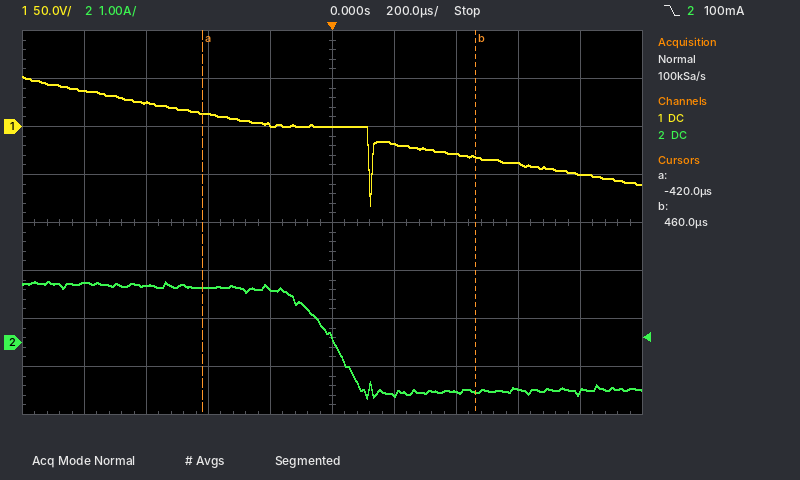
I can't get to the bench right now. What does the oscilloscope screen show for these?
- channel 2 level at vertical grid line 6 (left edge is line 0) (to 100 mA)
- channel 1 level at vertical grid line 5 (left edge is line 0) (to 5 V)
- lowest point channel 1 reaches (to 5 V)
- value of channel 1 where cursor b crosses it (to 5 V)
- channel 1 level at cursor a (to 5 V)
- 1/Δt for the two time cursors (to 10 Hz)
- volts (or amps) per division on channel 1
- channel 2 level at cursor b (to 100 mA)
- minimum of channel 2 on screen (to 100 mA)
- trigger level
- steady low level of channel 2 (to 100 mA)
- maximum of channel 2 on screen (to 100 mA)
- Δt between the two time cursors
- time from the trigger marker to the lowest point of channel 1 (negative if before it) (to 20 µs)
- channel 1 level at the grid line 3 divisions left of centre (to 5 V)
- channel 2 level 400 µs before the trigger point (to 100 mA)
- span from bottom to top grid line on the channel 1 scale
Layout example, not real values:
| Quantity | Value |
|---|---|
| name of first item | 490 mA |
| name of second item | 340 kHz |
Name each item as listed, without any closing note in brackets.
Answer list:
| Quantity | Value |
|---|---|
| channel 2 level at vertical grid line 6 (left edge is line 0) | -1.1 A |
| channel 1 level at vertical grid line 5 (left edge is line 0) | 0 V |
| lowest point channel 1 reaches | -80 V |
| value of channel 1 where cursor b crosses it | -30 V |
| channel 1 level at cursor a | 15 V |
| 1/Δt for the two time cursors | 1.14 kHz |
| volts (or amps) per division on channel 1 | 50 V |
| channel 2 level at cursor b | -1.0 A |
| minimum of channel 2 on screen | -1.2 A |
| trigger level | 100 mA |
| steady low level of channel 2 | -1.0 A |
| maximum of channel 2 on screen | 1.3 A |
| Δt between the two time cursors | 880 µs |
| time from the trigger marker to the lowest point of channel 1 (negative if before it) | +120 µs |
| channel 1 level at the grid line 3 divisions left of centre | 25 V |
| channel 2 level 400 µs before the trigger point | 1.1 A |
| span from bottom to top grid line on the channel 1 scale | 400 V |
